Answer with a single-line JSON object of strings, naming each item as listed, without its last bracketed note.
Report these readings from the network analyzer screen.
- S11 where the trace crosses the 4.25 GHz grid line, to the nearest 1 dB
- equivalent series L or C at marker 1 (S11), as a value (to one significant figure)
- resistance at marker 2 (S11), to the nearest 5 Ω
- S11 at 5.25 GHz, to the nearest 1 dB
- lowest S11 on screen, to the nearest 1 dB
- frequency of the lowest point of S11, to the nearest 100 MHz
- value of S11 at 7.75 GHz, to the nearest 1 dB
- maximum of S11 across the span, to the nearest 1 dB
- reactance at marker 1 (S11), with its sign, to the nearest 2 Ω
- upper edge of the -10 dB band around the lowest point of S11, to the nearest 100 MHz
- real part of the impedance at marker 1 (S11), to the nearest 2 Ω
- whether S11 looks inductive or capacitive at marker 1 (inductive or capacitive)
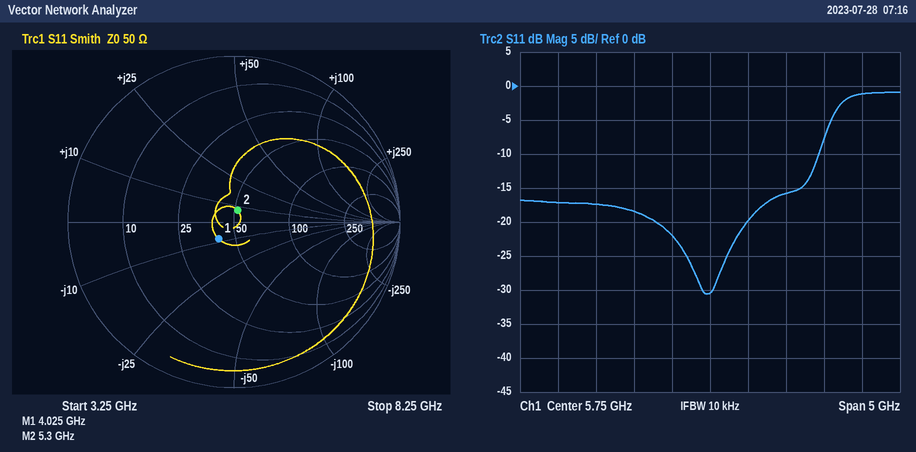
{"S11 where the trace crosses the 4.25 GHz grid line, to the nearest 1 dB": "-17 dB", "equivalent series L or C at marker 1 (S11), as a value": "5 pF", "resistance at marker 2 (S11), to the nearest 5 Ω": "50 Ω", "S11 at 5.25 GHz, to the nearest 1 dB": "-22 dB", "lowest S11 on screen, to the nearest 1 dB": "-31 dB", "frequency of the lowest point of S11, to the nearest 100 MHz": "5.7 GHz", "value of S11 at 7.75 GHz, to the nearest 1 dB": "-1 dB", "maximum of S11 across the span, to the nearest 1 dB": "-1 dB", "reactance at marker 1 (S11), with its sign, to the nearest 2 Ω": "-8 Ω", "upper edge of the -10 dB band around the lowest point of S11, to the nearest 100 MHz": "7.2 GHz", "real part of the impedance at marker 1 (S11), to the nearest 2 Ω": "40 Ω", "whether S11 looks inductive or capacitive at marker 1": "capacitive"}
